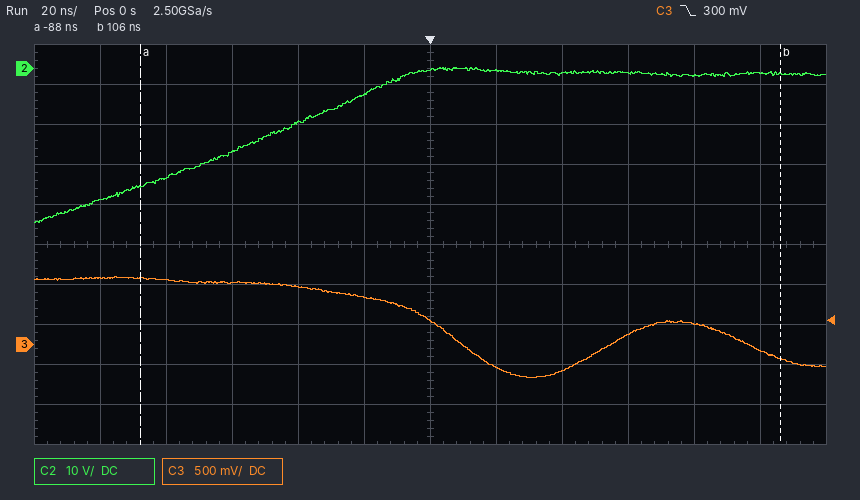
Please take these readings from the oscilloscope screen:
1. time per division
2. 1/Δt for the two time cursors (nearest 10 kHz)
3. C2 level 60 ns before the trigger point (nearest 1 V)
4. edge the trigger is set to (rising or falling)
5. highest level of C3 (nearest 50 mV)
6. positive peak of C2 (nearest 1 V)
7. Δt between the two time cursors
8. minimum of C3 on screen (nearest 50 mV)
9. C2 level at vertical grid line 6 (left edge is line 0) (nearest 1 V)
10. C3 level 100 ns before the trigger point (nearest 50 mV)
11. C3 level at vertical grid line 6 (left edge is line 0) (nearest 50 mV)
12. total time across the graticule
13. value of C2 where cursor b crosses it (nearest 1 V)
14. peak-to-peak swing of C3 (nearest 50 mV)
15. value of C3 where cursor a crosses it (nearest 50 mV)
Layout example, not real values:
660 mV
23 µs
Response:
20 ns
5.15 MHz
-21 V
falling
850 mV
0 V
194 ns
-400 mV
0 V
850 mV
300 mV
240 ns
-1 V
1.25 V
850 mV
